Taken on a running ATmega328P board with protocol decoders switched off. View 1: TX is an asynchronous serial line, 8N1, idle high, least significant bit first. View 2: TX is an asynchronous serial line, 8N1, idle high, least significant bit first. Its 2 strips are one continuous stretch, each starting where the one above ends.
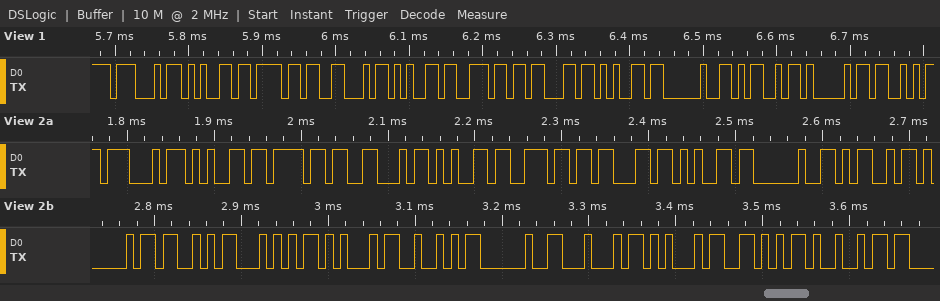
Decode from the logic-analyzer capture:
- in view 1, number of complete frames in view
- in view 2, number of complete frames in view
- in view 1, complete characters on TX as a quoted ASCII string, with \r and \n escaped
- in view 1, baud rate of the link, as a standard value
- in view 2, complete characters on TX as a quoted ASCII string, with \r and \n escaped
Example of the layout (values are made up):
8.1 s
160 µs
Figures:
12
20
"GeoFence MAS"
115200 baud
"GeoFence MASTER DEVI"
